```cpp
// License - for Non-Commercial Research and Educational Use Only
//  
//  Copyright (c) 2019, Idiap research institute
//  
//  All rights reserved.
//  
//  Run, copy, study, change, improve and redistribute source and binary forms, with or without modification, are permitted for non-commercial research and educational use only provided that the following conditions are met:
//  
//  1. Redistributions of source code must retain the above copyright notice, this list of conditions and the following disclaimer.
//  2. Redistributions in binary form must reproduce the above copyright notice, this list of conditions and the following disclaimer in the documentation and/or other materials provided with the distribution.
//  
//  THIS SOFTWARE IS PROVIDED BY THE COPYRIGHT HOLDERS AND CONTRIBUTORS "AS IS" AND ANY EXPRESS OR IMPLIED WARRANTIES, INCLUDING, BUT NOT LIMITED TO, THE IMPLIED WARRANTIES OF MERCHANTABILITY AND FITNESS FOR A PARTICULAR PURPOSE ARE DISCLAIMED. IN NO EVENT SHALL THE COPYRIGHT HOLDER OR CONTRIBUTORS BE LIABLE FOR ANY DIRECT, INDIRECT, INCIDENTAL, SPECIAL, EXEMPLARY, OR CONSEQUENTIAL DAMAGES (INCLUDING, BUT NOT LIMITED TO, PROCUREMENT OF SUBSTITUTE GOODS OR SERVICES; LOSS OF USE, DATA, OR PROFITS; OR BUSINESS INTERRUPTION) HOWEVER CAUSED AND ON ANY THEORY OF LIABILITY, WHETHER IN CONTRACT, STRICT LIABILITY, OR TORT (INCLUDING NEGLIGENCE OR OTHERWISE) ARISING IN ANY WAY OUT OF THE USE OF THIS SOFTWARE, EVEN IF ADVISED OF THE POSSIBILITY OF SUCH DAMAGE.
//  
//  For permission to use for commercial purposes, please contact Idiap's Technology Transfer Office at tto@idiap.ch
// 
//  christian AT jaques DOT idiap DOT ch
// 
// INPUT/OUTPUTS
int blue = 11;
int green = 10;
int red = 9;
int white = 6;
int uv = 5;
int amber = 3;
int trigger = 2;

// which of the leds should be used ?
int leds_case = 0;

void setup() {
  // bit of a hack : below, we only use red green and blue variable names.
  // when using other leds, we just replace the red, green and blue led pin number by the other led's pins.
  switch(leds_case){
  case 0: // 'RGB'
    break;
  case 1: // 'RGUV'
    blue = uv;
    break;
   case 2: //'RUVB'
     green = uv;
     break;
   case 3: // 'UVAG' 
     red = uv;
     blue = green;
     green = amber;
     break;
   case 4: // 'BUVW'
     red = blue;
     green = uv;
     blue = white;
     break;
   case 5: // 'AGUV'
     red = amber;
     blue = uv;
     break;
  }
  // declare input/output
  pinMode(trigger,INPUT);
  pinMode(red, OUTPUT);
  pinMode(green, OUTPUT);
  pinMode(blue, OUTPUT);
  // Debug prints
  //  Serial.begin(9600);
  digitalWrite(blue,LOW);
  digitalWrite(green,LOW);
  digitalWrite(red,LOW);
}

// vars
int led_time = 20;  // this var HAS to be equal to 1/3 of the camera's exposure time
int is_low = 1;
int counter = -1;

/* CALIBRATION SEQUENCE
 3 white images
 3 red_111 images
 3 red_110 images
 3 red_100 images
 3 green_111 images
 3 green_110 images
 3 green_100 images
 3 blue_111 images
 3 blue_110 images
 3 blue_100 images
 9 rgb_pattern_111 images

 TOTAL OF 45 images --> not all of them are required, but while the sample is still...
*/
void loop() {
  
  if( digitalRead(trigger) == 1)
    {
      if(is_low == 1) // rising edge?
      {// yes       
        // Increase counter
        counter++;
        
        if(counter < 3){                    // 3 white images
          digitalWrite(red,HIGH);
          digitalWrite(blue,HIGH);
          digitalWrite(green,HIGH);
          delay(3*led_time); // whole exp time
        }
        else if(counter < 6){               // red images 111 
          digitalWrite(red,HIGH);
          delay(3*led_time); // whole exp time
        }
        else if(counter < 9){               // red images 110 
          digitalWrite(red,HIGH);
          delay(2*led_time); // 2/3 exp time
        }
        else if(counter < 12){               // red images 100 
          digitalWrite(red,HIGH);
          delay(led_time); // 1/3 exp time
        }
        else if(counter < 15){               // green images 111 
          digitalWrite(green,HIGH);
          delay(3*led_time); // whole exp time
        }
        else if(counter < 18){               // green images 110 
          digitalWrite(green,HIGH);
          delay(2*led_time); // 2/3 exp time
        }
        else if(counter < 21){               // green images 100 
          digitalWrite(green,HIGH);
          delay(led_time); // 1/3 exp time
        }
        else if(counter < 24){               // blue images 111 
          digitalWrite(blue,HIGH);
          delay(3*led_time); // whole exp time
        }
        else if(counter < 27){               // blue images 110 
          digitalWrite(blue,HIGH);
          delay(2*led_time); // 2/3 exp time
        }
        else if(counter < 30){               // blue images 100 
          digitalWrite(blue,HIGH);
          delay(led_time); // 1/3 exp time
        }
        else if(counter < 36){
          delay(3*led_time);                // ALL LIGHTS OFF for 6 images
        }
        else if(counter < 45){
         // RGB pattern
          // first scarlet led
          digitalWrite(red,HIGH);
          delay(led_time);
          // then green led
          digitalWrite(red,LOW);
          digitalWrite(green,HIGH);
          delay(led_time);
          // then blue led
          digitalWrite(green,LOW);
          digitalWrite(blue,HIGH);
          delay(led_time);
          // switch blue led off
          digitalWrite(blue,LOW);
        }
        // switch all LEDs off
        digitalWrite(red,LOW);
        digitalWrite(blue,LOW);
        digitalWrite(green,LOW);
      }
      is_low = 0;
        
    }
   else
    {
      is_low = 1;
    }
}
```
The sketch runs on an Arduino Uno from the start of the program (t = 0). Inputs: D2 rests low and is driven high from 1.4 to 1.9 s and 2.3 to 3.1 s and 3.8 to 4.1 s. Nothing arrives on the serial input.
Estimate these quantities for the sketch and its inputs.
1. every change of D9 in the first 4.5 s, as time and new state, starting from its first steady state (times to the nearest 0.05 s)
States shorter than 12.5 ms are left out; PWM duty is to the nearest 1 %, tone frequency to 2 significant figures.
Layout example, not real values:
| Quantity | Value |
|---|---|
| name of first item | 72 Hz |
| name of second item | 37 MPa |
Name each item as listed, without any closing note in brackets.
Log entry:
| Quantity | Value |
|---|---|
| every change of D9 in the first 4.5 s, as time and new state, starting from its first steady state | 0 s low; 1.4 s high; 1.45 s low; 2.3 s high; 2.35 s low; 3.8 s high; 3.85 s low |
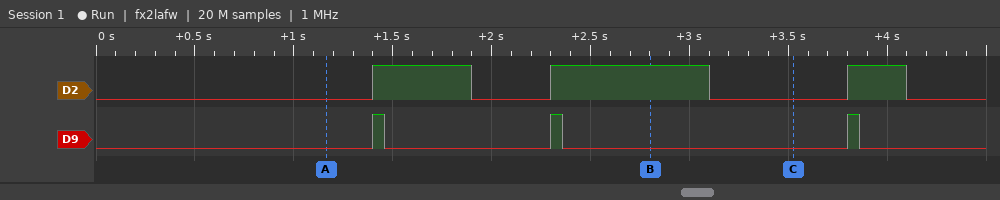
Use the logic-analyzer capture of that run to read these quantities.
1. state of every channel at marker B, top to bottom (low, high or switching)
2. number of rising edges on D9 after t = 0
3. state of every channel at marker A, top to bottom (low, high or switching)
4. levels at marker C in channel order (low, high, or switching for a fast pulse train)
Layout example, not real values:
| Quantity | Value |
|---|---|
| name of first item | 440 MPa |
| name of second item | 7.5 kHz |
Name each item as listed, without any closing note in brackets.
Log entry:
| Quantity | Value |
|---|---|
| state of every channel at marker B, top to bottom | D2 high, D9 low |
| number of rising edges on D9 after t = 0 | 3 |
| state of every channel at marker A, top to bottom | D2 low, D9 low |
| levels at marker C in channel order | D2 low, D9 low |
